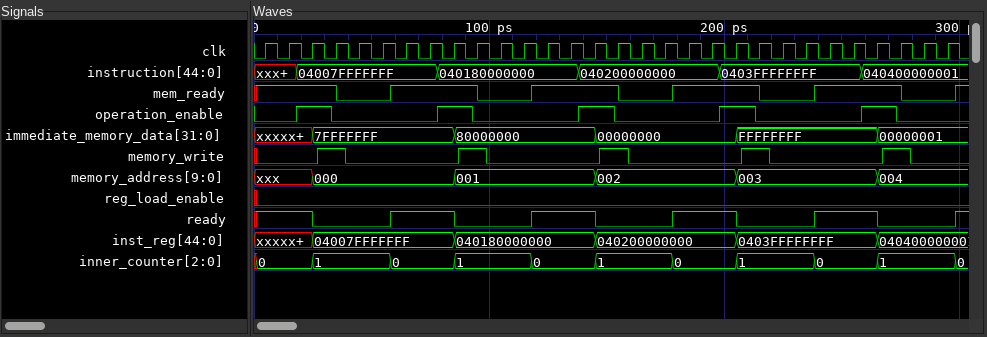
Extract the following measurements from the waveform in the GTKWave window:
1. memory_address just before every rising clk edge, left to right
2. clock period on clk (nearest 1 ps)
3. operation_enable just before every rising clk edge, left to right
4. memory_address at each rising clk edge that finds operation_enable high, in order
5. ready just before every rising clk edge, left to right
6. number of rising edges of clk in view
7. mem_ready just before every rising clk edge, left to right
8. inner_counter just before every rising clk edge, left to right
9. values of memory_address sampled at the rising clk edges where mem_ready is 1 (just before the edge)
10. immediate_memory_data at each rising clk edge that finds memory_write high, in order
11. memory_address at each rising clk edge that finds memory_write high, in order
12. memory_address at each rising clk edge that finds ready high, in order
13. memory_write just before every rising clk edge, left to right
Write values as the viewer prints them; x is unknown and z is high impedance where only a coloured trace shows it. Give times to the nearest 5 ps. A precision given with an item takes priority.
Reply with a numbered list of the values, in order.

1. xxx, xxx, xxx, 000, 000, 000, 000, 000, 000, 001, 001, 001, 001, 001, 001, 002, 002, 002, 002, 002, 002, 003, 003, 003, 003, 003, 003, 004, 004, 004
2. 10 ps
3. 0 0 1 0 0 0 0 0 1 0 0 0 0 0 1 0 0 0 0 0 1 0 0 0 0 0 1 0 0 0
4. xxx, 000, 001, 002, 003
5. 1 1 1 0 0 0 1 1 1 0 0 0 1 1 1 0 0 0 1 1 1 0 0 0 1 1 1 0 0 0
6. 30
7. 1 1 1 1 0 0 1 1 1 1 0 0 1 1 1 1 0 0 1 1 1 1 0 0 1 1 1 1 0 0
8. 0, 0, 0, 1, 1, 1, 0, 0, 0, 1, 1, 1, 0, 0, 0, 1, 1, 1, 0, 0, 0, 1, 1, 1, 0, 0, 0, 1, 1, 1
9. xxx, xxx, xxx, 000, 000, 000, 000, 001, 001, 001, 001, 002, 002, 002, 002, 003, 003, 003, 003, 004
10. 7FFFFFFF, 80000000, 00000000, FFFFFFFF, 00000001
11. 000, 001, 002, 003, 004
12. xxx, xxx, xxx, 000, 000, 000, 001, 001, 001, 002, 002, 002, 003, 003, 003
13. 0 0 0 1 0 0 0 0 0 1 0 0 0 0 0 1 0 0 0 0 0 1 0 0 0 0 0 1 0 0
